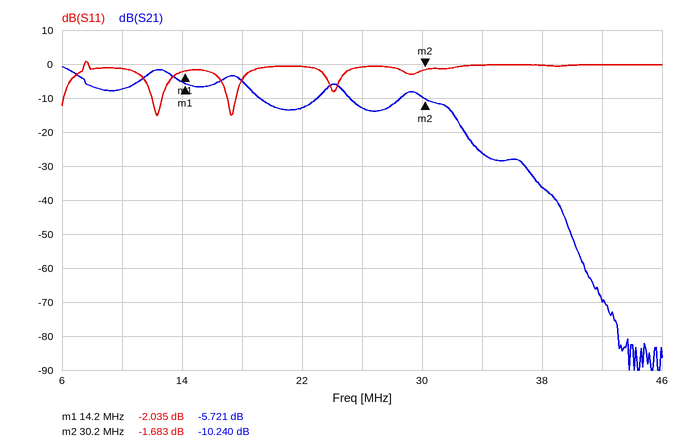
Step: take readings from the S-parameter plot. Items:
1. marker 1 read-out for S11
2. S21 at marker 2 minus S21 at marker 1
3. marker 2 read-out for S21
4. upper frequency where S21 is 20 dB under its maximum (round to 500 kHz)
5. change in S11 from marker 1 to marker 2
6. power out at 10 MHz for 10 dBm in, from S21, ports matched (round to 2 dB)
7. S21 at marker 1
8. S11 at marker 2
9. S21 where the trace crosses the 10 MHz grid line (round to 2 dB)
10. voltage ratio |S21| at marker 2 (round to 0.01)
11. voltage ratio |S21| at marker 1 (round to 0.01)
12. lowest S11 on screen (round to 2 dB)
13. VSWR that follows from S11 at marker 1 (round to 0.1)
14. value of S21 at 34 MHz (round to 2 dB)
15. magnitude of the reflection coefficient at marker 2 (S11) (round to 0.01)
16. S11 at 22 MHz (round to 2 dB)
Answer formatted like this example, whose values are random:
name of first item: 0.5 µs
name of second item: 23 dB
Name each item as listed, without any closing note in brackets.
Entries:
marker 1 read-out for S11: -2.035 dB
S21 at marker 2 minus S21 at marker 1: -4.519 dB
marker 2 read-out for S21: -10.240 dB
upper frequency where S21 is 20 dB under its maximum: 33.0 MHz
change in S11 from marker 1 to marker 2: 0.352 dB
power out at 10 MHz for 10 dBm in, from S21, ports matched: 2 dBm
S21 at marker 1: -5.721 dB
S11 at marker 2: -1.683 dB
S21 where the trace crosses the 10 MHz grid line: -8 dB
voltage ratio |S21| at marker 2: 0.31
voltage ratio |S21| at marker 1: 0.52
lowest S11 on screen: -16 dB
VSWR that follows from S11 at marker 1: 8.6
value of S21 at 34 MHz: -26 dB
magnitude of the reflection coefficient at marker 2 (S11): 0.82
S11 at 22 MHz: 0 dB
